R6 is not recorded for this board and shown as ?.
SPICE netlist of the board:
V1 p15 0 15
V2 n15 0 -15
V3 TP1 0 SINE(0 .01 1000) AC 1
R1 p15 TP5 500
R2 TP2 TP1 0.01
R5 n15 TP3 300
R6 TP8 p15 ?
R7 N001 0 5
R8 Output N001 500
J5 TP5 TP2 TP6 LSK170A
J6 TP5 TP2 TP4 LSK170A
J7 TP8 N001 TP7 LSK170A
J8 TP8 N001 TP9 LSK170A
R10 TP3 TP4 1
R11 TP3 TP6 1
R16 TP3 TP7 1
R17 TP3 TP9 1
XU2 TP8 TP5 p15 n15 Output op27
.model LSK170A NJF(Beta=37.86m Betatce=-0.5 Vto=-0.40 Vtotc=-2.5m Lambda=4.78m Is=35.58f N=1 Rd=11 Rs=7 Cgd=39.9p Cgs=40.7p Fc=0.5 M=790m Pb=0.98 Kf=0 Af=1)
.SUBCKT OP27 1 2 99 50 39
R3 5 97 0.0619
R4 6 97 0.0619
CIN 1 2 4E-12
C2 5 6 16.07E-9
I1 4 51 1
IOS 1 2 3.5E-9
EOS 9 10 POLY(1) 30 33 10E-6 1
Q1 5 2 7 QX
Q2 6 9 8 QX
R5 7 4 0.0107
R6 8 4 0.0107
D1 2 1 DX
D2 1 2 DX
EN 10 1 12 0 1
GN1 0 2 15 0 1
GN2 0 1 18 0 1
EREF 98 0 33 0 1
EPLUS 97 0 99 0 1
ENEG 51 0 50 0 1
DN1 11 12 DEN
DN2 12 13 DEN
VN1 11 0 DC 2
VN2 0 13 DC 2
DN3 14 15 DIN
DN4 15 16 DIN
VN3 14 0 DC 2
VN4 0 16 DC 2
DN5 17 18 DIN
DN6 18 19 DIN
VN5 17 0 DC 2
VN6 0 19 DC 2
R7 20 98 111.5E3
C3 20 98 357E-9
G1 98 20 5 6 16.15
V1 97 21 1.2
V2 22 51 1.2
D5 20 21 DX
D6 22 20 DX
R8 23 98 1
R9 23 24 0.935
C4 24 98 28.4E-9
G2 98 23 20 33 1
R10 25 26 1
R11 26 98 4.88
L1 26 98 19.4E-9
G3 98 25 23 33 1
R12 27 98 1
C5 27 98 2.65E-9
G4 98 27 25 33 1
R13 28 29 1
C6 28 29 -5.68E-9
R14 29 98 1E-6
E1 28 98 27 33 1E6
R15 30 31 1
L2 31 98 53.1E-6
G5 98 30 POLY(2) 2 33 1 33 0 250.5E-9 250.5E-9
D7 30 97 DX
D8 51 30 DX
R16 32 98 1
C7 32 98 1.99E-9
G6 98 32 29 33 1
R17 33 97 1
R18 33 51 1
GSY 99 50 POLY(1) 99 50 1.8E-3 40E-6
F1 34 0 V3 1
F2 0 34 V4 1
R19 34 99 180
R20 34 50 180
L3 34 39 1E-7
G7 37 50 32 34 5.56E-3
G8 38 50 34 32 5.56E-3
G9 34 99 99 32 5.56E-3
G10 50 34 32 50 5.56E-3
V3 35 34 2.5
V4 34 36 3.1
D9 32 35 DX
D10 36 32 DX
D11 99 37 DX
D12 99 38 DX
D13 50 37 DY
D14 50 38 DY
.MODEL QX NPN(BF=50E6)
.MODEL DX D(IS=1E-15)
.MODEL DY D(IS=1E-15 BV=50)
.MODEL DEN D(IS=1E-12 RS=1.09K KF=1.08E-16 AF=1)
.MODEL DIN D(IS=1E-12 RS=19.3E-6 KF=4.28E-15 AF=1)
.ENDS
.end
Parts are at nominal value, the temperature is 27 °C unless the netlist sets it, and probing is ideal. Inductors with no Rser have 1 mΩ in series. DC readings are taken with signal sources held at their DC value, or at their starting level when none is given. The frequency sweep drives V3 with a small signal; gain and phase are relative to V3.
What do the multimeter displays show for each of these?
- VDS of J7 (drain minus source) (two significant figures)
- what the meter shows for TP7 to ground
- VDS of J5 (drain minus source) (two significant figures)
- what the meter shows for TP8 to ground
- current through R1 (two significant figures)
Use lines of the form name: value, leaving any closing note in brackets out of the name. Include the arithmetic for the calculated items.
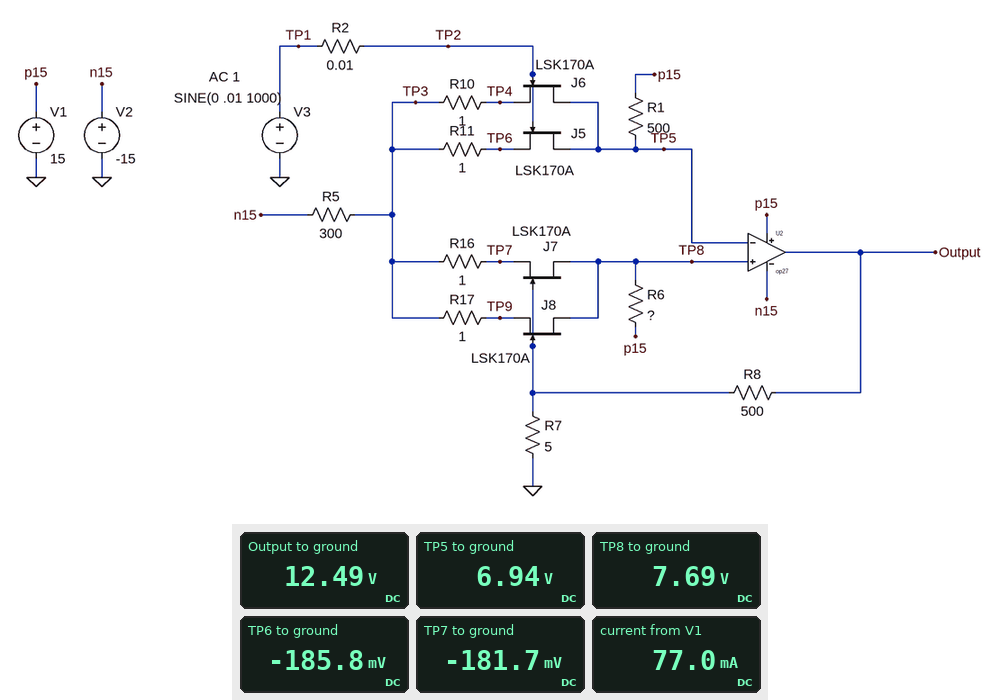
VDS of J7 (drain minus source): 7.69 V - (-181.7 mV) = 7.9 V
what the meter shows for TP7 to ground: -181.7 mV
VDS of J5 (drain minus source): 6.94 V - (-185.8 mV) = 7.1 V
what the meter shows for TP8 to ground: 7.69 V
current through R1: (15 V - 6.94 V) / 500 Ω = 16 mA
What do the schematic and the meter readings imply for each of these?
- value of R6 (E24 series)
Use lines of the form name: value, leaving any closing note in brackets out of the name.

value of R6: 220 Ω
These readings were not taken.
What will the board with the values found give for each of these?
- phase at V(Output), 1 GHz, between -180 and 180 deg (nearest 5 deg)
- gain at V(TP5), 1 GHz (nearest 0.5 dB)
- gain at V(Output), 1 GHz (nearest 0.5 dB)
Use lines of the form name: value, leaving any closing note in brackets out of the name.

phase at V(Output), 1 GHz, between -180 and 180 deg: 50 deg
gain at V(TP5), 1 GHz: -2.0 dB
gain at V(Output), 1 GHz: -9.5 dB
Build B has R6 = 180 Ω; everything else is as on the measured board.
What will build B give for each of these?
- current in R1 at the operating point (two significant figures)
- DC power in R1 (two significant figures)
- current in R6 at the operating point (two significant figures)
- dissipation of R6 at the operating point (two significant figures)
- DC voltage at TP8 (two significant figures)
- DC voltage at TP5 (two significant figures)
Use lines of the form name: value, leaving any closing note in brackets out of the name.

current in R1 at the operating point: 14 mA
DC power in R1: 100 mW
current in R6 at the operating point: 35 mA
dissipation of R6 at the operating point: 220 mW
DC voltage at TP8: 8.7 V
DC voltage at TP5: 7.9 V
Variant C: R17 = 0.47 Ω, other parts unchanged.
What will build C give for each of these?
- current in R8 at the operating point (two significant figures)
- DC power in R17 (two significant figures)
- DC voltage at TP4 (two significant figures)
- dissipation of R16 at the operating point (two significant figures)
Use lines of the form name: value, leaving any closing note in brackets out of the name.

current in R8 at the operating point: 25 mA
DC power in R17: 100 µW
DC voltage at TP4: -180 mV
dissipation of R16 at the operating point: 200 µW
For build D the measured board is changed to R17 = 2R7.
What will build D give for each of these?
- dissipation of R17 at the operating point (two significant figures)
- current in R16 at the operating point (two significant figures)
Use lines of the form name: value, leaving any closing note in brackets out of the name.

dissipation of R17 at the operating point: 510 µW
current in R16 at the operating point: 15 mA
